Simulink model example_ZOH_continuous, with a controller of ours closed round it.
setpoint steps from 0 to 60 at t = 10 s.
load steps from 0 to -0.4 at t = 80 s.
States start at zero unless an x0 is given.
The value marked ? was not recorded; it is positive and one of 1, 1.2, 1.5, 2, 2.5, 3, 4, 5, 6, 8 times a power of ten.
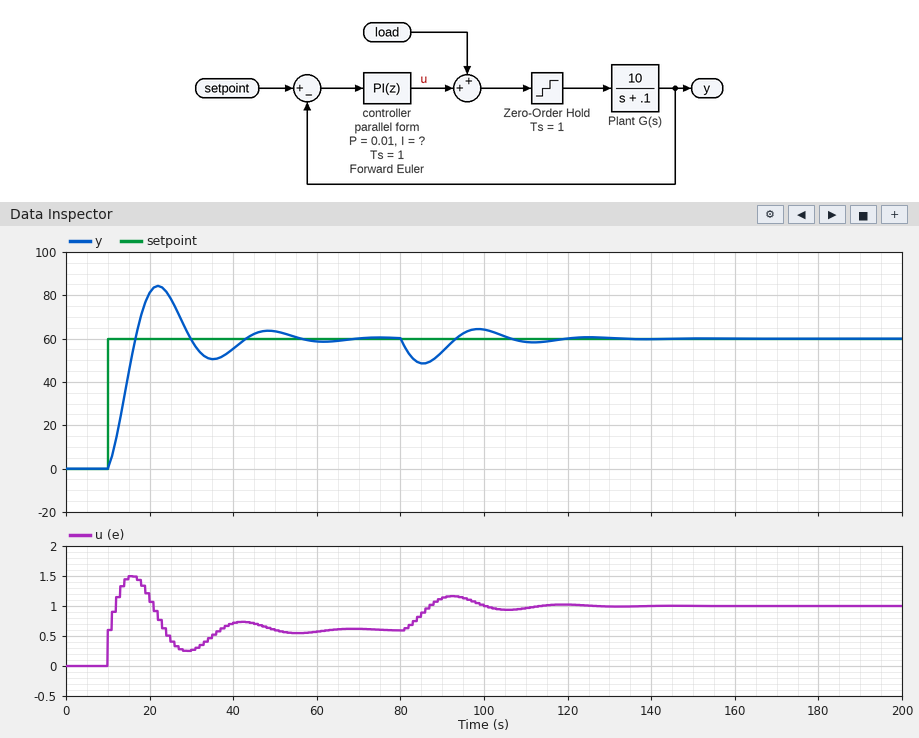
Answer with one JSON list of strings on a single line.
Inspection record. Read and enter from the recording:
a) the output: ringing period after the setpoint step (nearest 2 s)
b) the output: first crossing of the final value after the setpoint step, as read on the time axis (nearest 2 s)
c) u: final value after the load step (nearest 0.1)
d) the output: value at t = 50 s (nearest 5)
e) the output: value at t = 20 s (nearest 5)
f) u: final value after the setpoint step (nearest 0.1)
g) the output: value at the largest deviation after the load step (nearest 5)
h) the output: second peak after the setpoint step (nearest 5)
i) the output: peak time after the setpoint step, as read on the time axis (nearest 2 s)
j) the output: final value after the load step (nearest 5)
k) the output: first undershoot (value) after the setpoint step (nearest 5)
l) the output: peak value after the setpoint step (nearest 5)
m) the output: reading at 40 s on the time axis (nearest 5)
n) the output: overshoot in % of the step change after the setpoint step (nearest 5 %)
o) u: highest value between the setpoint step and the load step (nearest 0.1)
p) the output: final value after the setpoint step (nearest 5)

["26 s", "16 s", "1.0", "65", "80", "0.6", "50", "65", "22 s", "60", "50", "85", "55", "40 %", "1.5", "60"]
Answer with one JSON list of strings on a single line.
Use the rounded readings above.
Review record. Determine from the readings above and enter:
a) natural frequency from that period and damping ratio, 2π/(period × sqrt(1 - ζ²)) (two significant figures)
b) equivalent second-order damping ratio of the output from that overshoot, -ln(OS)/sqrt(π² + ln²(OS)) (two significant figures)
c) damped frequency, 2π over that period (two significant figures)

["0.25 rad/s", "0.28", "0.24 rad/s"]
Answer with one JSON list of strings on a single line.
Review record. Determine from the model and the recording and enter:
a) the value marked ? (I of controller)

["0.006"]
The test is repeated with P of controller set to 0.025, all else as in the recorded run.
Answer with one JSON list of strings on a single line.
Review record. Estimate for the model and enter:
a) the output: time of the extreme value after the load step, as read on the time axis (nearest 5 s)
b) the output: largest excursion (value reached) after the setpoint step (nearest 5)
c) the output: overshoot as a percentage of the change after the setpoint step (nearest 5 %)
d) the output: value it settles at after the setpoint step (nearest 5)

["85 s", "70", "15 %", "60"]
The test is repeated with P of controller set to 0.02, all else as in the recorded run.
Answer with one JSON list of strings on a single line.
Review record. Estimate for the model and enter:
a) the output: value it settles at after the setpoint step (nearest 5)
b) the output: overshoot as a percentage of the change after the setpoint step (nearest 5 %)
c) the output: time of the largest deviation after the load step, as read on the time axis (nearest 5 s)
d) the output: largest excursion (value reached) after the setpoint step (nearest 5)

["60", "20 %", "85 s", "75"]
